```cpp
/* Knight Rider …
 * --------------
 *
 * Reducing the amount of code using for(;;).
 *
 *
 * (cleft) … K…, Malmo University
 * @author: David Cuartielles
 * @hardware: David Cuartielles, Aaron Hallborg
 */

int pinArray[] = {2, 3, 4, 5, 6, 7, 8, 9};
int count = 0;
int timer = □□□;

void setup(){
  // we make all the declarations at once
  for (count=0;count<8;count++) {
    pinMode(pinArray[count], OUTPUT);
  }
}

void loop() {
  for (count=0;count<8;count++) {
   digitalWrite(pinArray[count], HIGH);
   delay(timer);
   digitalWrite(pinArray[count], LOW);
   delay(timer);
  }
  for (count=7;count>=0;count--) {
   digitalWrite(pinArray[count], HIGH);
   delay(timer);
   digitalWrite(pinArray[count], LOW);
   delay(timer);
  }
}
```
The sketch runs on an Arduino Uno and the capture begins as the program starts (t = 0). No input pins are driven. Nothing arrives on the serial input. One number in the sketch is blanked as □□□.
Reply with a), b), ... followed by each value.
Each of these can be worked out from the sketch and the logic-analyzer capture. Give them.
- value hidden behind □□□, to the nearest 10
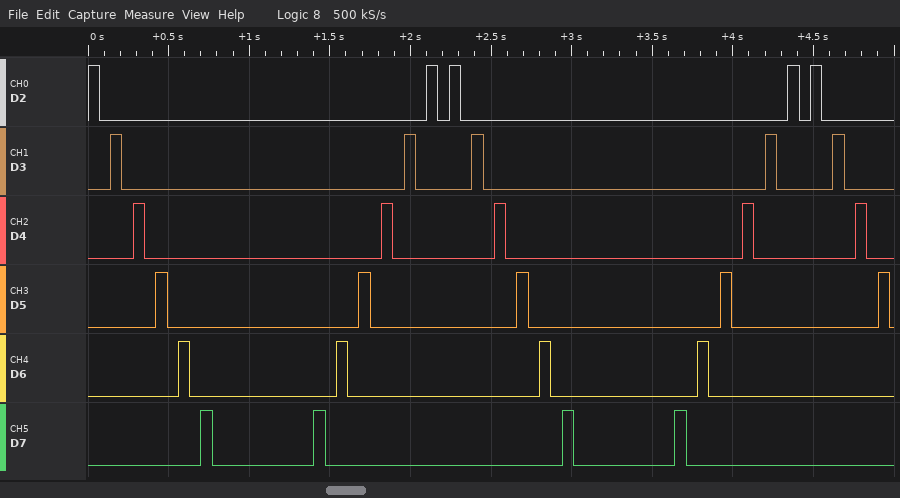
a) 70
